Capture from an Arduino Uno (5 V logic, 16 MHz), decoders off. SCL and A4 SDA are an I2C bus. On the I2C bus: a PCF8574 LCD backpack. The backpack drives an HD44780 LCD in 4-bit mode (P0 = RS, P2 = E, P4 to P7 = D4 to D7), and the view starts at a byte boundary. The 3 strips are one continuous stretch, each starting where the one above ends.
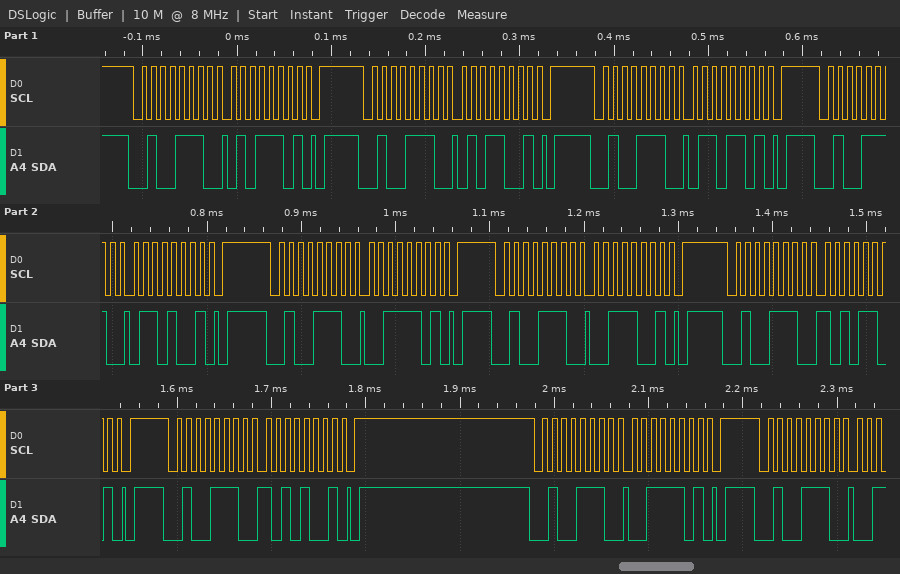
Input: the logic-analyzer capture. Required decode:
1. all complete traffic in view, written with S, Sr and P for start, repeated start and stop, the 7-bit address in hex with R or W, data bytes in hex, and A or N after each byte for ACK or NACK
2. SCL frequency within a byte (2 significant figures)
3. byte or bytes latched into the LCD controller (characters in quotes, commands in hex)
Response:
S 27W A 5D A P S 27W A 59 A P S 27W A 6D A P S 27W A 69 A P S 27W A 3D A P S 27W A 39 A P S 27W A AD A P S 27W A A9 A P S 27W A 3D A P S 27W A
100 kHz
'V' ':'
